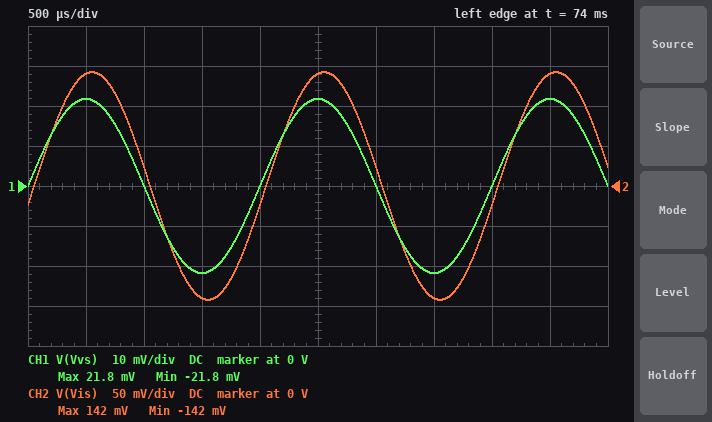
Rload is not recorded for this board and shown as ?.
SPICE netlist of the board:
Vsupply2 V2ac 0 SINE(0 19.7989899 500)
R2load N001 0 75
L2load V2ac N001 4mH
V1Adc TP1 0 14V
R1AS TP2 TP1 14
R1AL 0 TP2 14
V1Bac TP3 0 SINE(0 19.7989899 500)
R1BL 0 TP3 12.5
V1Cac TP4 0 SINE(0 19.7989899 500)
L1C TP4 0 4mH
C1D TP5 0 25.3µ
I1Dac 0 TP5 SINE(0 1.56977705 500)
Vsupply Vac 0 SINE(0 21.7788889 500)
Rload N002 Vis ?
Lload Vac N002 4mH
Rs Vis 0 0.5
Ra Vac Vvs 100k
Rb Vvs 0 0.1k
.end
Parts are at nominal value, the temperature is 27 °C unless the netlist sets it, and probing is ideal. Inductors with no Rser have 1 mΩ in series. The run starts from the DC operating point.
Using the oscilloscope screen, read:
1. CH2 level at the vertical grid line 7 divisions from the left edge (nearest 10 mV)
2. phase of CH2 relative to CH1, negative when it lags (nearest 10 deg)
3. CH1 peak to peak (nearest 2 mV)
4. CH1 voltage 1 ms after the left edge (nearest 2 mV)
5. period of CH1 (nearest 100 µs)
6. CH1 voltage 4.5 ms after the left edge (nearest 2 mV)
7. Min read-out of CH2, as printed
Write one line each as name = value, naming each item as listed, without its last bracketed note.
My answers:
CH2 level at the vertical grid line 7 divisions from the left edge = -140 mV
phase of CH2 relative to CH1, negative when it lags = -10 deg
CH1 peak to peak = 44 mV
CH1 voltage 1 ms after the left edge = 0 V
period of CH1 = 2.0 ms
CH1 voltage 4.5 ms after the left edge = 22 mV
Min read-out of CH2, as printed = -142 mV
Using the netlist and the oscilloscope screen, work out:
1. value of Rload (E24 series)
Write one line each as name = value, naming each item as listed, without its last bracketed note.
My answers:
value of Rload = 75 Ω
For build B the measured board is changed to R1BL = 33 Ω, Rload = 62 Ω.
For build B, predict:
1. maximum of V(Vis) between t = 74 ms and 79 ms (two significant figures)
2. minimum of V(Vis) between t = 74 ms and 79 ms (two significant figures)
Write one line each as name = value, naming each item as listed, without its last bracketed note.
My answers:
maximum of V(Vis) between t = 74 ms and 79 ms = 170 mV
minimum of V(Vis) between t = 74 ms and 79 ms = -170 mV
